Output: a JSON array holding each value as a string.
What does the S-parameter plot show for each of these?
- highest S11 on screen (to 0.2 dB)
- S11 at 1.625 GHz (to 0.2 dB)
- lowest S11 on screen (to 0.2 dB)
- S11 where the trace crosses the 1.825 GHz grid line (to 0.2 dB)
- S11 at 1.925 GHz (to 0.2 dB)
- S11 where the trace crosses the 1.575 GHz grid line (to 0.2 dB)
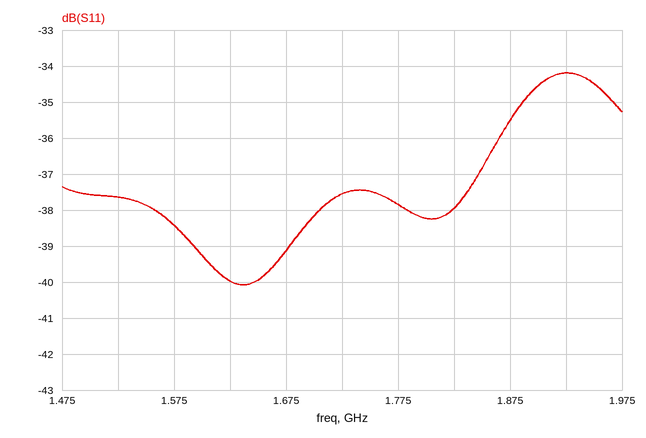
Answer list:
["-34.2 dB", "-40.0 dB", "-40.0 dB", "-38.0 dB", "-34.2 dB", "-38.4 dB"]
